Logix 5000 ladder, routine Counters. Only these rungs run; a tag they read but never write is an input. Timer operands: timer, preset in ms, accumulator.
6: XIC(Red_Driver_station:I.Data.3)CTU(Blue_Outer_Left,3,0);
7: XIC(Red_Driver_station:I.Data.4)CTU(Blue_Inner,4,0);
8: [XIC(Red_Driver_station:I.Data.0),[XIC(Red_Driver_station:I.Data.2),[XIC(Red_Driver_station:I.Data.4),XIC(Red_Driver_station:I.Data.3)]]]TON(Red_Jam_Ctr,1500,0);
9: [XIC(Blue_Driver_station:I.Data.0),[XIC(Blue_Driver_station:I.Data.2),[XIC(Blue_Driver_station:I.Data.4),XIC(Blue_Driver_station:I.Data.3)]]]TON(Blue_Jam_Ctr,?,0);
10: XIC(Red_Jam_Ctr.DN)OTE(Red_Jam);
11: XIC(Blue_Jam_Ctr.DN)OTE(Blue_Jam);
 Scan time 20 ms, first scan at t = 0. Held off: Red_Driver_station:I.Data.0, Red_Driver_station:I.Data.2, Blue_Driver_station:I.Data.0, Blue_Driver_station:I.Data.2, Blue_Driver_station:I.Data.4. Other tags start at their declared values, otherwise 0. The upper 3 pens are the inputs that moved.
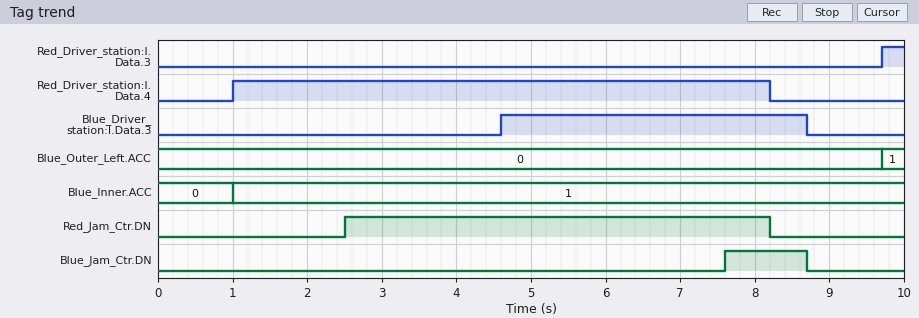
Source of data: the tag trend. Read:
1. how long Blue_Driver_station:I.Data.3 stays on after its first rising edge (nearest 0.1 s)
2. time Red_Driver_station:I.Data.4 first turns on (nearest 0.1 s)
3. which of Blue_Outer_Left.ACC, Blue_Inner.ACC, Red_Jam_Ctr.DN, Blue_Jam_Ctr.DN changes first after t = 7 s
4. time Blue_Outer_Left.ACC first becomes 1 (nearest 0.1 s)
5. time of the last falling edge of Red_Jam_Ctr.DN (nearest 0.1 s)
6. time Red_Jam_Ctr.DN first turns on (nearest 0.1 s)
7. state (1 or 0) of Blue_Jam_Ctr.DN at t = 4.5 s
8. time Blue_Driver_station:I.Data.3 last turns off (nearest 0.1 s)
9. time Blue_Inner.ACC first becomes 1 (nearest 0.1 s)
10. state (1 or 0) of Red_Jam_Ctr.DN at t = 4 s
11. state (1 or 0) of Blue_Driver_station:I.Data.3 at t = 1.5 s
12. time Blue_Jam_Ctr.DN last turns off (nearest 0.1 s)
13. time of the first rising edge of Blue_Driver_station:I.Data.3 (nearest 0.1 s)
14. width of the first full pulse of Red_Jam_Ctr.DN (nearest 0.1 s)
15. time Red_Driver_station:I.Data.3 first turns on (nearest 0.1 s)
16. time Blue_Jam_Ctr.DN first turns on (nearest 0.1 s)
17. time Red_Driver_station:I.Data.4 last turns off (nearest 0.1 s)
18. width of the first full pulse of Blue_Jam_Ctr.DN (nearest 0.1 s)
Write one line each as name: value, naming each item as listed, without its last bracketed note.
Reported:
how long Blue_Driver_station:I.Data.3 stays on after its first rising edge: 4.1 s
time Red_Driver_station:I.Data.4 first turns on: 1.0 s
which of Blue_Outer_Left.ACC, Blue_Inner.ACC, Red_Jam_Ctr.DN, Blue_Jam_Ctr.DN changes first after t = 7 s: Blue_Jam_Ctr.DN
time Blue_Outer_Left.ACC first becomes 1: 9.7 s
time of the last falling edge of Red_Jam_Ctr.DN: 8.2 s
time Red_Jam_Ctr.DN first turns on: 2.5 s
state (1 or 0) of Blue_Jam_Ctr.DN at t = 4.5 s: 0
time Blue_Driver_station:I.Data.3 last turns off: 8.7 s
time Blue_Inner.ACC first becomes 1: 1.0 s
state (1 or 0) of Red_Jam_Ctr.DN at t = 4 s: 1
state (1 or 0) of Blue_Driver_station:I.Data.3 at t = 1.5 s: 0
time Blue_Jam_Ctr.DN last turns off: 8.7 s
time of the first rising edge of Blue_Driver_station:I.Data.3: 4.6 s
width of the first full pulse of Red_Jam_Ctr.DN: 5.7 s
time Red_Driver_station:I.Data.3 first turns on: 9.7 s
time Blue_Jam_Ctr.DN first turns on: 7.6 s
time Red_Driver_station:I.Data.4 last turns off: 8.2 s
width of the first full pulse of Blue_Jam_Ctr.DN: 1.1 s
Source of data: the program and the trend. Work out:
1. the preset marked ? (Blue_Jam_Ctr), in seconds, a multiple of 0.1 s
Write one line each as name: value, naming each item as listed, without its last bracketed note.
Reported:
the preset marked ? (Blue_Jam_Ctr), in seconds, a multiple of 0.1 s: 3.0 s
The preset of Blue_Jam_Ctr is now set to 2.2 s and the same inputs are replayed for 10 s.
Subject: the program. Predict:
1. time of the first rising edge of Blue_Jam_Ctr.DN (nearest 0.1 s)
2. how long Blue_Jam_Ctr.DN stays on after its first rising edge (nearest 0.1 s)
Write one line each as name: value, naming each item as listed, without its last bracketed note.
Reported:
time of the first rising edge of Blue_Jam_Ctr.DN: 6.8 s
how long Blue_Jam_Ctr.DN stays on after its first rising edge: 1.9 s
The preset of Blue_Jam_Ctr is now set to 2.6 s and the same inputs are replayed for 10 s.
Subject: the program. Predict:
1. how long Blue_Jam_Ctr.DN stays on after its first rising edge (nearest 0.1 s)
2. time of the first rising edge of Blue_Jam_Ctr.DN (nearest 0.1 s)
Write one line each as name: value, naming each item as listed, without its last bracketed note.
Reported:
how long Blue_Jam_Ctr.DN stays on after its first rising edge: 1.5 s
time of the first rising edge of Blue_Jam_Ctr.DN: 7.2 s
